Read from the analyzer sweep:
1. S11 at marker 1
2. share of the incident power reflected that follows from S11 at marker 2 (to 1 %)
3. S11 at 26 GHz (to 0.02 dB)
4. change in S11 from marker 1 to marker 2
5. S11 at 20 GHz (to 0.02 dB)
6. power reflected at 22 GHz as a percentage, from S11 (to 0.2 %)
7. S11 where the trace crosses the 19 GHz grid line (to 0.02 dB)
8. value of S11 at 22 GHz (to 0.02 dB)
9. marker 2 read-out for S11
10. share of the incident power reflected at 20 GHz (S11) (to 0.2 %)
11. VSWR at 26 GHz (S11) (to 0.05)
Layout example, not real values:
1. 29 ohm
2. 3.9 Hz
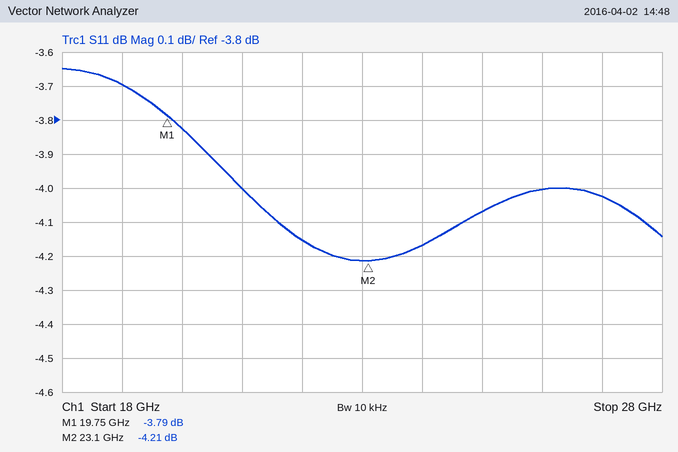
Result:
1. -3.79 dB
2. 38 %
3. -4.00 dB
4. -0.42 dB
5. -3.82 dB
6. 38.4 %
7. -3.70 dB
8. -4.16 dB
9. -4.21 dB
10. 41.4 %
11. 4.40
